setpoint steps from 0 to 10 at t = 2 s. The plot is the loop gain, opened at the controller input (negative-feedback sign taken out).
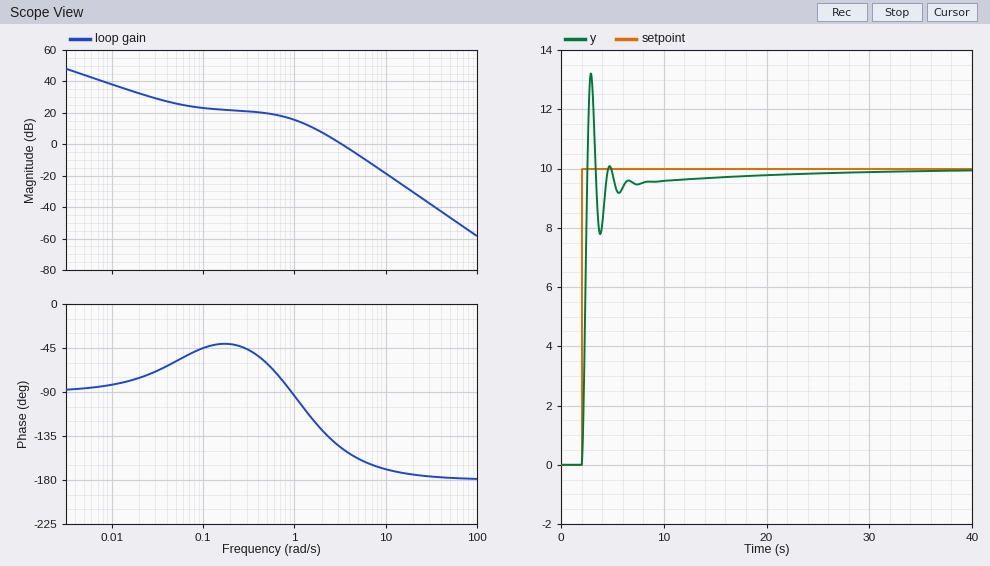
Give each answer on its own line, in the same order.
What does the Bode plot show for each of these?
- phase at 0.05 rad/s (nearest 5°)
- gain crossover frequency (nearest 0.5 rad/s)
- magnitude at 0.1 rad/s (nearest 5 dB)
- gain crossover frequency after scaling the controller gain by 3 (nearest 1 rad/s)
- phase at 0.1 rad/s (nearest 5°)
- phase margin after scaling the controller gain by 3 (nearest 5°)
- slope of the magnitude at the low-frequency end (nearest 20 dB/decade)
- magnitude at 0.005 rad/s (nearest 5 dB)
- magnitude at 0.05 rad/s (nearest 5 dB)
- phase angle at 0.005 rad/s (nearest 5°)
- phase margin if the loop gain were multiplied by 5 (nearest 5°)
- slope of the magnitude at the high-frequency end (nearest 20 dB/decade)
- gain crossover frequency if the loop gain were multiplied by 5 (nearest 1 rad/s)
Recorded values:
-60°
3.5 rad/s
25 dB
6 rad/s
-45°
20°
-20 dB/decade
45 dB
25 dB
-85°
15°
-40 dB/decade
8 rad/s
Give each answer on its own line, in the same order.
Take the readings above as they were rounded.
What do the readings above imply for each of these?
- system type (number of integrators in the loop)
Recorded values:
1
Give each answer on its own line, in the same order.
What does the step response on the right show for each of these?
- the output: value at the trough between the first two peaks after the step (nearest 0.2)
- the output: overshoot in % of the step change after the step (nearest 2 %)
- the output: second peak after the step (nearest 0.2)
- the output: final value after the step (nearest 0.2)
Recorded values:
7.8
32 %
10.0
10.0
